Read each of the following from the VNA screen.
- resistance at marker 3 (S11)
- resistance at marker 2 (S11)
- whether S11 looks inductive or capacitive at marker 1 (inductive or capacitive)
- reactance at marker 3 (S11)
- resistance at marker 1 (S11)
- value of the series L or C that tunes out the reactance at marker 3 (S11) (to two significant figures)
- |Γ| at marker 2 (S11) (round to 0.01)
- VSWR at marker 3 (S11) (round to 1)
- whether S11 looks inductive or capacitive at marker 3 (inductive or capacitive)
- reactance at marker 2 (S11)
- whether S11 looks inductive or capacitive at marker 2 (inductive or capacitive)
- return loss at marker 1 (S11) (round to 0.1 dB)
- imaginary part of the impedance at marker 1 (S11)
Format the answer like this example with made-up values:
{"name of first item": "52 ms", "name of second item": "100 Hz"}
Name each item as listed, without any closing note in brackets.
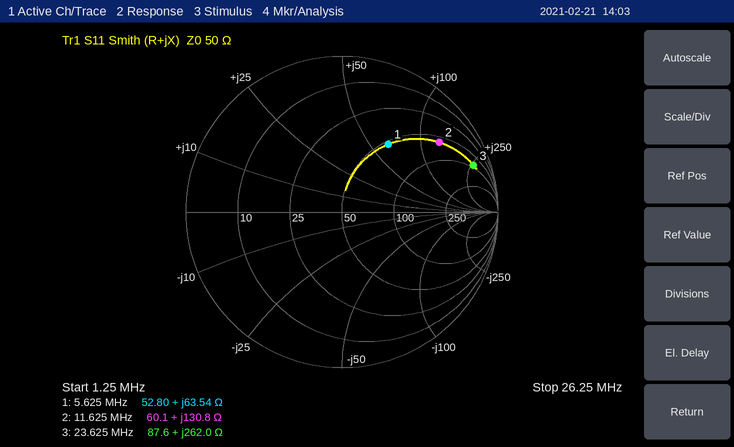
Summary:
{"resistance at marker 3": "87.6 Ω", "resistance at marker 2": "60.1 Ω", "whether S11 looks inductive or capacitive at marker 1": "inductive", "reactance at marker 3": "+262.0 Ω", "resistance at marker 1": "52.80 Ω", "value of the series L or C that tunes out the reactance at marker 3 (S11)": "26 pF", "|Γ| at marker 2 (S11)": "0.77", "VSWR at marker 3 (S11)": "18", "whether S11 looks inductive or capacitive at marker 3": "inductive", "reactance at marker 2": "+130.8 Ω", "whether S11 looks inductive or capacitive at marker 2": "inductive", "return loss at marker 1 (S11)": "5.6 dB", "imaginary part of the impedance at marker 1": "+63.54 Ω"}
